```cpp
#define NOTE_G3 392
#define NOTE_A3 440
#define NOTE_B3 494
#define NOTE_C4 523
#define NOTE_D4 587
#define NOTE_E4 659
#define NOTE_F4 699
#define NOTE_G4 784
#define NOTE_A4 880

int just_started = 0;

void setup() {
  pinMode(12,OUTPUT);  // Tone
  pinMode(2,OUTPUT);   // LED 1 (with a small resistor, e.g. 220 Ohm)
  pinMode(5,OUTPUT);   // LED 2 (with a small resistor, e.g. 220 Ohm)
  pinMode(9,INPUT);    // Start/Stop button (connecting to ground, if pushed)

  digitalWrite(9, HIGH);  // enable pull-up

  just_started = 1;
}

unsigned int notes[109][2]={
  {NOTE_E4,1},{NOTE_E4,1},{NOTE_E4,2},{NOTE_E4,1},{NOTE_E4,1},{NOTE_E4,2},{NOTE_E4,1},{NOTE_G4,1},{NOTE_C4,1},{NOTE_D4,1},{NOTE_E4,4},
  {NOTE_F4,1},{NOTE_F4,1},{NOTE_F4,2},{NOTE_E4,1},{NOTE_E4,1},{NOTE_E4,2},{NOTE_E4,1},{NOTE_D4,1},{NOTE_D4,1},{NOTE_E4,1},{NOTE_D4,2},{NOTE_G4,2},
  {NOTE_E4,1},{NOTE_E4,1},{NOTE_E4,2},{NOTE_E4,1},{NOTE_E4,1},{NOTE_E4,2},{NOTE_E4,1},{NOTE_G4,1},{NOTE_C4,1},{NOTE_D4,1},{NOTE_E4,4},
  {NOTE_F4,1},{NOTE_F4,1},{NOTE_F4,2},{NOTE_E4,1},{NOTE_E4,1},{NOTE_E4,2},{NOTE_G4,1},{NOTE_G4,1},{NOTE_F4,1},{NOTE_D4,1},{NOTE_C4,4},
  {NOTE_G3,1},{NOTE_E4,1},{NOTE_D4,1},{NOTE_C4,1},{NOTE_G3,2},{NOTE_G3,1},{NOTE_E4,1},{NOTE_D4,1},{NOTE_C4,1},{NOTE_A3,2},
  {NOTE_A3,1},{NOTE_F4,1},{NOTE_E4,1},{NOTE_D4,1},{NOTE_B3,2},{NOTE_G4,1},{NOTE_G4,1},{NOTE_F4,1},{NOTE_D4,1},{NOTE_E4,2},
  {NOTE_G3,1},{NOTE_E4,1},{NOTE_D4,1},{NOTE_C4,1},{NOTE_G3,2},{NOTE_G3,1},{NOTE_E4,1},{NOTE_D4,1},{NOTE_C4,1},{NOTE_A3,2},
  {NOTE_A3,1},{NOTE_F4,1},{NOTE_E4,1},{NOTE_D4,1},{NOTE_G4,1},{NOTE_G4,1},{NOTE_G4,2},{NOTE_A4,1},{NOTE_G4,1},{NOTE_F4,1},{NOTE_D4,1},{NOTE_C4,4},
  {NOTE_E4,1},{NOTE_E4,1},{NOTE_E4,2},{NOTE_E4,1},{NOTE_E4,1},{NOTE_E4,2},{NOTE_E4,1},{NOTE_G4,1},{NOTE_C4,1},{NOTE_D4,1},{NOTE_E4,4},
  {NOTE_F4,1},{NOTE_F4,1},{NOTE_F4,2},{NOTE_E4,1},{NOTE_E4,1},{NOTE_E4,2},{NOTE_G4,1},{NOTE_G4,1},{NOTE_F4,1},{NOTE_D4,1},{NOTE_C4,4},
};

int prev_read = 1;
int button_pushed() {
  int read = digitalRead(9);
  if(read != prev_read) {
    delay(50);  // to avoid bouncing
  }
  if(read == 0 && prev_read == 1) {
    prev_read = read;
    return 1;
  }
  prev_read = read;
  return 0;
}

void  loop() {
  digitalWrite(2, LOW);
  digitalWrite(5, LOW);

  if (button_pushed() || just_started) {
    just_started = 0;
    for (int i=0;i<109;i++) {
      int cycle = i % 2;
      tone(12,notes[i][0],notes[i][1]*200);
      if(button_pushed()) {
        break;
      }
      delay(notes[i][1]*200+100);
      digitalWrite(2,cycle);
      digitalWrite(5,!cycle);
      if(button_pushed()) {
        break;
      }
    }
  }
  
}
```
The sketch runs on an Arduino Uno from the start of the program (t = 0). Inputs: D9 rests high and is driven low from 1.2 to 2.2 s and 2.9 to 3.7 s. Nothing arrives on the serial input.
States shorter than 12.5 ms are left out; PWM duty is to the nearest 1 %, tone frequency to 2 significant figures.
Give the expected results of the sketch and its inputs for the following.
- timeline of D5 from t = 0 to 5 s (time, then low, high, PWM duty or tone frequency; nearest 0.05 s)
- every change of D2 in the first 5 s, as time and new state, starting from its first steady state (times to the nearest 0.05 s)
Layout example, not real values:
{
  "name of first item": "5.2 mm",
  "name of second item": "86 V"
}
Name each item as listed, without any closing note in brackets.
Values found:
{
  "timeline of D5 from t = 0 to 5 s": "0 s low; 0.3 s high; 0.6 s low; 1.1 s high; 1.4 s low; 3.25 s high; 3.55 s low; 4.05 s high; 4.4 s low; 4.7 s high",
  "every change of D2 in the first 5 s, as time and new state, starting from its first steady state": "0 s low; 0.6 s high; 1.1 s low; 1.4 s high; 1.45 s low; 3.55 s high; 4.05 s low; 4.4 s high; 4.7 s low"
}
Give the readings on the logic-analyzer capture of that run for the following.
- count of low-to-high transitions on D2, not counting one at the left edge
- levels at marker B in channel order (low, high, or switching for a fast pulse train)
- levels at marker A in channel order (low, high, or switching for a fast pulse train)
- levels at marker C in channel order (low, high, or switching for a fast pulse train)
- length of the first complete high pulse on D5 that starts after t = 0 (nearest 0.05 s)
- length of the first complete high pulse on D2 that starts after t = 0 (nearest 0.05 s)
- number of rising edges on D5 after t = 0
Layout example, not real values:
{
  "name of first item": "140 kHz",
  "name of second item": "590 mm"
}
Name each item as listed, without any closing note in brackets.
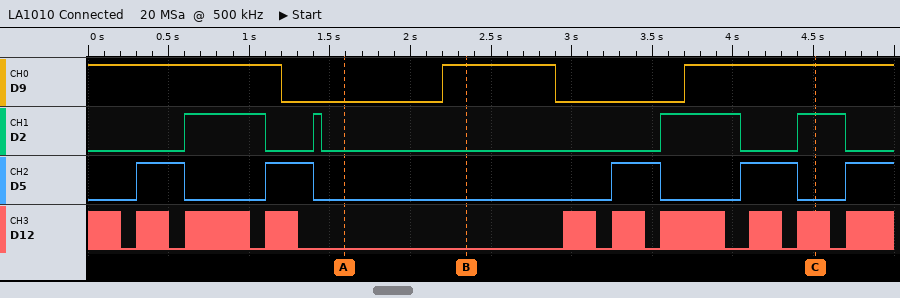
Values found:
{
  "count of low-to-high transitions on D2, not counting one at the left edge": "4",
  "levels at marker B in channel order": "D9 high, D2 low, D5 low, D12 low",
  "levels at marker A in channel order": "D9 low, D2 low, D5 low, D12 low",
  "levels at marker C in channel order": "D9 high, D2 high, D5 low, D12 switching",
  "length of the first complete high pulse on D5 that starts after t = 0": "0.30 s",
  "length of the first complete high pulse on D2 that starts after t = 0": "0.50 s",
  "number of rising edges on D5 after t = 0": "5"
}
